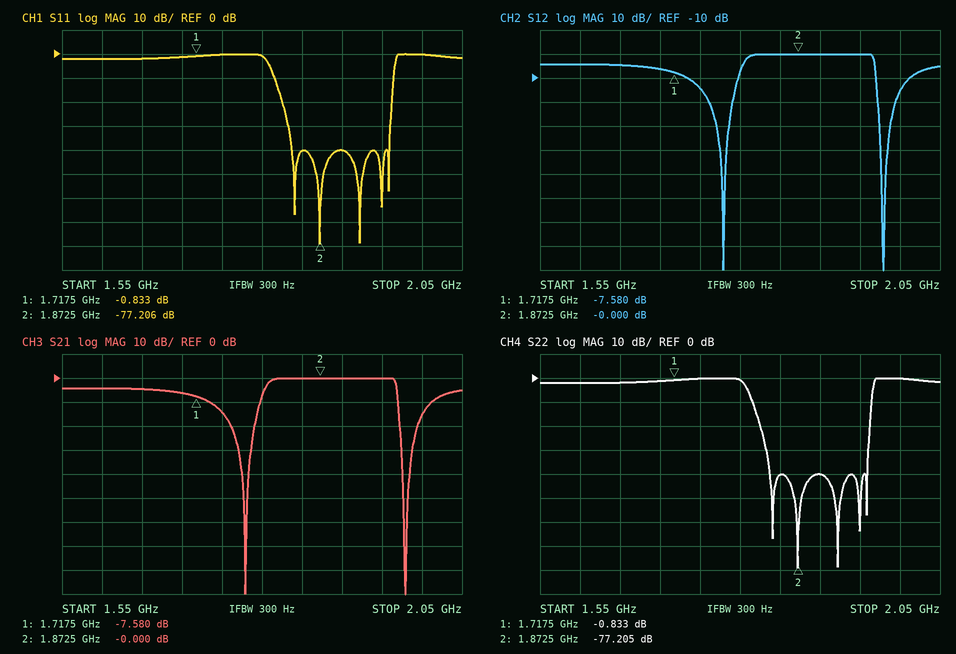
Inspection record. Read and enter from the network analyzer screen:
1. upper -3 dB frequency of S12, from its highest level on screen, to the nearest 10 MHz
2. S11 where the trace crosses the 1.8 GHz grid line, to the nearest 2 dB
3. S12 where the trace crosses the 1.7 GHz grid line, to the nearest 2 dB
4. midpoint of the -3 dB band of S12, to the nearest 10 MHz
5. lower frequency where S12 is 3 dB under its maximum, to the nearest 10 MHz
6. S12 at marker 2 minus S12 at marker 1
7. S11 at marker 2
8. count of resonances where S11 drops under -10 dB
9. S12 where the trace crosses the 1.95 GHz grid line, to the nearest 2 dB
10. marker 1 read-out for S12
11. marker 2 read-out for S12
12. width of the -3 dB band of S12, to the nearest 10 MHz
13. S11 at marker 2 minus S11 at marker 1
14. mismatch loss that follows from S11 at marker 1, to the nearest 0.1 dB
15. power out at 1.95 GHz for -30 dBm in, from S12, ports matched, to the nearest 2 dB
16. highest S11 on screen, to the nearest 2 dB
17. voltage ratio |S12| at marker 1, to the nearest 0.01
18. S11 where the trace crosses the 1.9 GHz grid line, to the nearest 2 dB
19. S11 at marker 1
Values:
1.97 GHz
0 dB
-6 dB
1.89 GHz
1.81 GHz
7.580 dB
-77.206 dB
5
0 dB
-7.580 dB
-0.000 dB
160 MHz
-76.373 dB
7.6 dB
-30 dBm
0 dB
0.42
-40 dB
-0.833 dB
